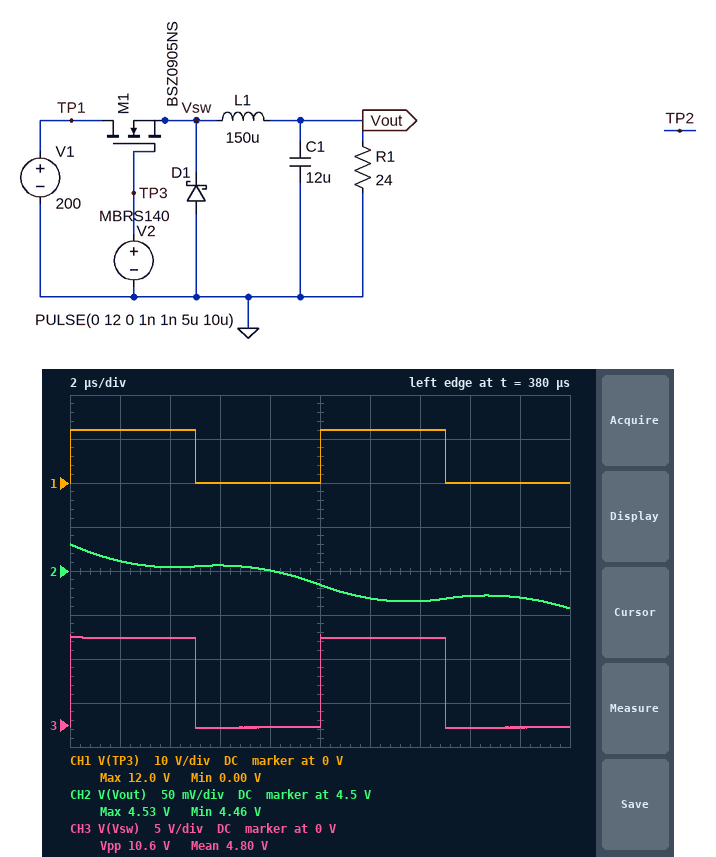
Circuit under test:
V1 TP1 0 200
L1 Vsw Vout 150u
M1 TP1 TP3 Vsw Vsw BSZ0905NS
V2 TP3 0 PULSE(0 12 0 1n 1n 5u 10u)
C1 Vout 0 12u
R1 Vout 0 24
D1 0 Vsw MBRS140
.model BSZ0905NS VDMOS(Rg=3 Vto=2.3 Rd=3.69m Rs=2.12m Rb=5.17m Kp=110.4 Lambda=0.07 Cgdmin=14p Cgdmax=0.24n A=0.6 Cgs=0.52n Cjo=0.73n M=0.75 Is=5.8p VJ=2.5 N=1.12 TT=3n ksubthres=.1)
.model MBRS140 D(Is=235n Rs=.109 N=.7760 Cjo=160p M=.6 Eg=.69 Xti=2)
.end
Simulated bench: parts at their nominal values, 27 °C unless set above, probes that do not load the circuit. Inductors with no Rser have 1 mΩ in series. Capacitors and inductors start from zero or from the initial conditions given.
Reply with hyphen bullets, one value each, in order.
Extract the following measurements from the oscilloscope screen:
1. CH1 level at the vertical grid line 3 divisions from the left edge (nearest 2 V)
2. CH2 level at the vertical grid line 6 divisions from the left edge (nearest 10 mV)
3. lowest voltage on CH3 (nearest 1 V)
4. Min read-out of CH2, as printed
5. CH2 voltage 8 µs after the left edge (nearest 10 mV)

- 0 V
- 4.47 V
- 0 V
- 4.46 V
- 4.50 V
